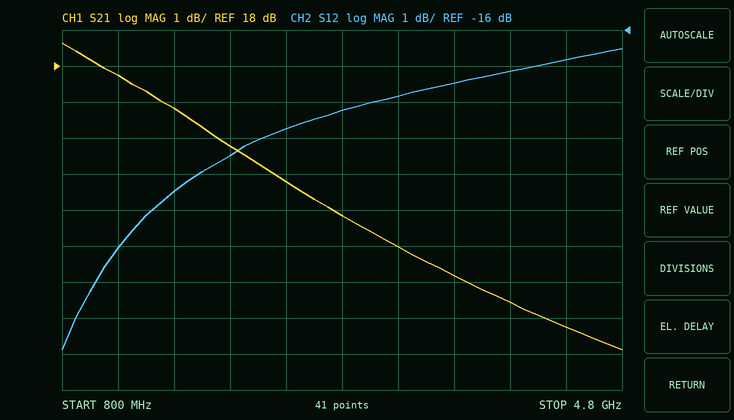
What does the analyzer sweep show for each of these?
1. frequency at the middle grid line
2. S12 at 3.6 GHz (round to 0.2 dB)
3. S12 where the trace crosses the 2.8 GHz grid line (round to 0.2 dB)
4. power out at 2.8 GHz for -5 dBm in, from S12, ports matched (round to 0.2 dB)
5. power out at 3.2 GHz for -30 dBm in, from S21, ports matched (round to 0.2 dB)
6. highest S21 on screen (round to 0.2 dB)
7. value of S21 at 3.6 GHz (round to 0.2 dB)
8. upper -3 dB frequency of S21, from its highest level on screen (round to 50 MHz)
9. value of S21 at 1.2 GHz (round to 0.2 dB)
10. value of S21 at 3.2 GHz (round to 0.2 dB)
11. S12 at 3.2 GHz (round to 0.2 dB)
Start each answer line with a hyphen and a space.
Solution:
- 2.8 GHz
- -17.4 dB
- -18.2 dB
- -23.2 dBm
- -17.0 dBm
- 18.6 dB
- 12.2 dB
- 2.05 GHz
- 17.8 dB
- 13.0 dB
- -17.8 dB
